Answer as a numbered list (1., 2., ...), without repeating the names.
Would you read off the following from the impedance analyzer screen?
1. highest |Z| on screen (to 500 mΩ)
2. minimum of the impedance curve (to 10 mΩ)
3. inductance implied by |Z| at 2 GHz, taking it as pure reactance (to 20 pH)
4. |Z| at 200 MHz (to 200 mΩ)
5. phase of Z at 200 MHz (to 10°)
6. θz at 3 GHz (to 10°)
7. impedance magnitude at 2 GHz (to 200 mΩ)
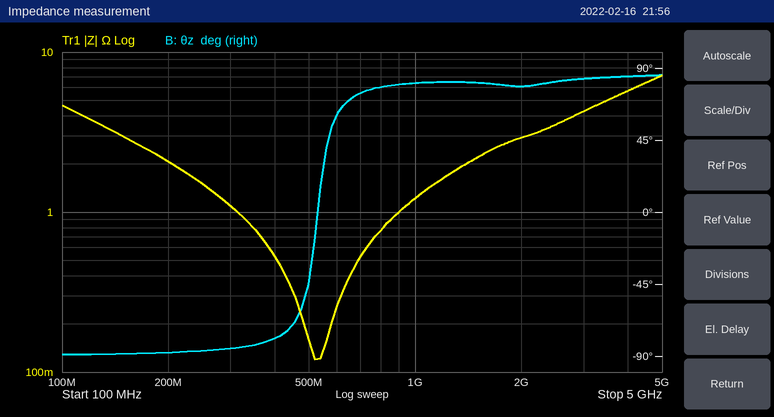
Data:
1. 7.0 Ω
2. 120 mΩ
3. 240 pH
4. 2.0 Ω
5. -90°
6. 80°
7. 3.0 Ω
